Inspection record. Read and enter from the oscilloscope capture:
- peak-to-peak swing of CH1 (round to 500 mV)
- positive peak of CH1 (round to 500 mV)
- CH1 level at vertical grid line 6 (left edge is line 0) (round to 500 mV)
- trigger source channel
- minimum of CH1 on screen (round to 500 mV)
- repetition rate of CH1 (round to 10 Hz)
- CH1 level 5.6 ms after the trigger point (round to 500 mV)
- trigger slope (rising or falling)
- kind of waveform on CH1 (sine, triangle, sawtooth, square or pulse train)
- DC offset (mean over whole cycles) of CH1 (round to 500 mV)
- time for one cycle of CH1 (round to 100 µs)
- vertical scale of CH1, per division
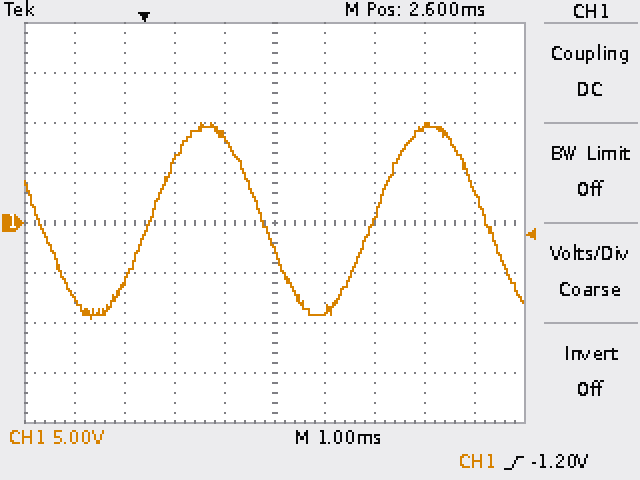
19.5 V
10.0 V
-8.5 V
CH1
-9.5 V
220 Hz
9.5 V
rising
sine
500 mV
4.5 ms
5 V
